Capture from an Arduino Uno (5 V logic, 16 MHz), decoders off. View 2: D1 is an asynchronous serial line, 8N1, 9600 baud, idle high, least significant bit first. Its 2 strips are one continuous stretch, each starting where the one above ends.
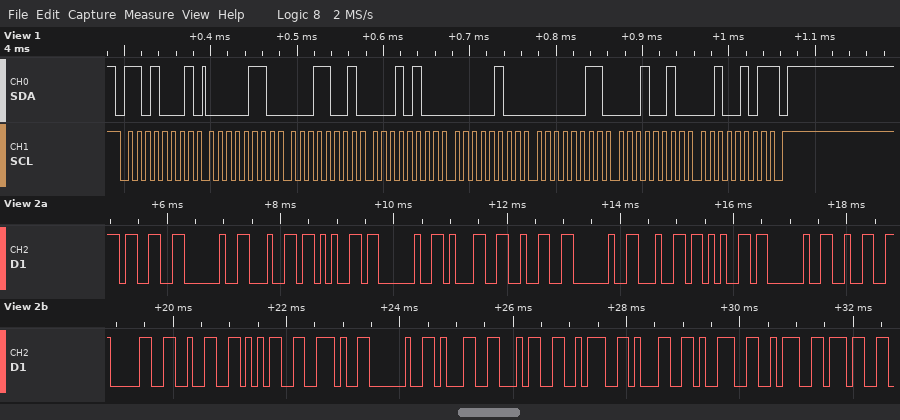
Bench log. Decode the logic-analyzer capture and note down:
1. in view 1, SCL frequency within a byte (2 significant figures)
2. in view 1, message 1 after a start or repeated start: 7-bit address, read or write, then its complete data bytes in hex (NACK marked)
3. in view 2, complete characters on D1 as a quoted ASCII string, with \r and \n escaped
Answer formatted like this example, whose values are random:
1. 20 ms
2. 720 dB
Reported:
1. 100 kHz
2. 0x68 read: 06 19 14 04 03 12 25 NACK
3. "3 de 12 de 2025. 14:19:7"
